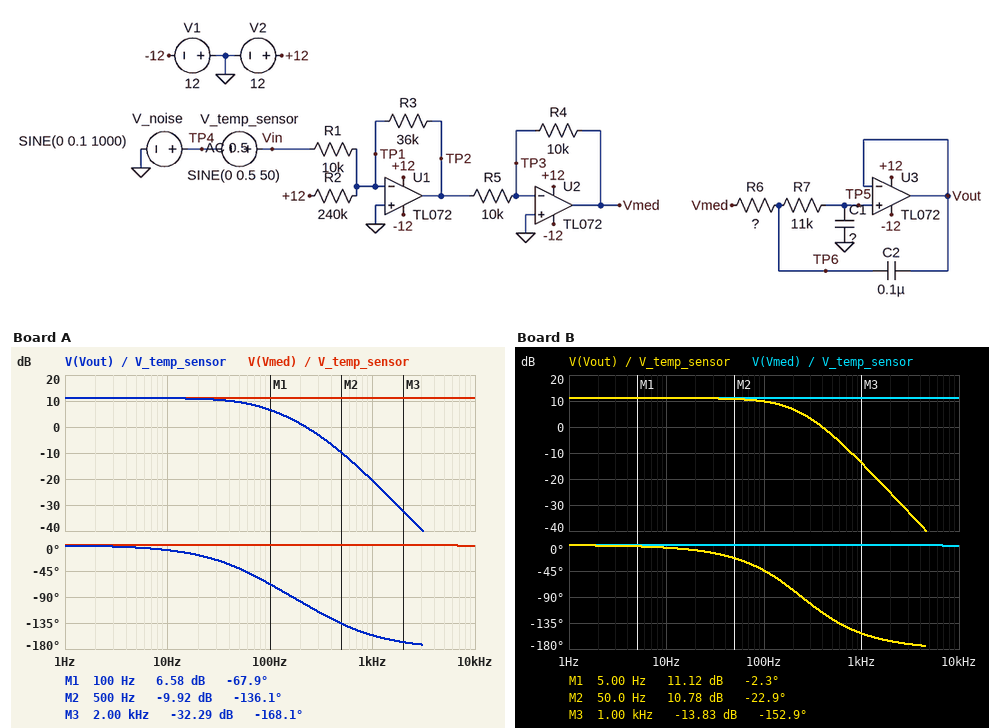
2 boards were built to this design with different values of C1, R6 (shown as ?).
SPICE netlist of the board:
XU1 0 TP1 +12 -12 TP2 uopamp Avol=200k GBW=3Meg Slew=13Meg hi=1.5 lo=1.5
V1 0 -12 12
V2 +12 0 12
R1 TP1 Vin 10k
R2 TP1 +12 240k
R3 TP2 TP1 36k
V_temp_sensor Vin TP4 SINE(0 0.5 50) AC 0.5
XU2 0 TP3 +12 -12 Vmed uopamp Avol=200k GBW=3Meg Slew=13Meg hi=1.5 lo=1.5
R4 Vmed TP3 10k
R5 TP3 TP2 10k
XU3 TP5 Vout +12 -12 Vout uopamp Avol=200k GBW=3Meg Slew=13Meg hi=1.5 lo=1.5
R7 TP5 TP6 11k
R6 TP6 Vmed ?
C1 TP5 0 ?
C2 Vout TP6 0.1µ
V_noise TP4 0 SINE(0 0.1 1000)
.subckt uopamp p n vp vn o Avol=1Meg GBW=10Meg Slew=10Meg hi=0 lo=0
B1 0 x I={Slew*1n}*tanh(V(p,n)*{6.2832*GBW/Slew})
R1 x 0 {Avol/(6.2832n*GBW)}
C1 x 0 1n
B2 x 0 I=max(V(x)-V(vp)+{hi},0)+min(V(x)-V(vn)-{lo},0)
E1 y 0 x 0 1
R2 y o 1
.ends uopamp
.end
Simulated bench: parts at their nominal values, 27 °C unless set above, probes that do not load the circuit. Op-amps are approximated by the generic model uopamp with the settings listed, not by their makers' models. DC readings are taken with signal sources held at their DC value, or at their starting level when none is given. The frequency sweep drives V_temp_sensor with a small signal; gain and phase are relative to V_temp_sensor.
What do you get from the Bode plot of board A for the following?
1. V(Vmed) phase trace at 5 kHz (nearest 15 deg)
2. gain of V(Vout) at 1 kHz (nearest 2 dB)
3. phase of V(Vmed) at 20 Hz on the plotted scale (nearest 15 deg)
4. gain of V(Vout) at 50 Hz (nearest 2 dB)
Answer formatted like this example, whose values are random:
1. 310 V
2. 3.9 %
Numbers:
1. 0 deg
2. -20 dB
3. 0 deg
4. 10 dB
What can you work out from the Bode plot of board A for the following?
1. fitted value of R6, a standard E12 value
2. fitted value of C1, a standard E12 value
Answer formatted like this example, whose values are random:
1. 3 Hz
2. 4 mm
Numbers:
1. 5.6 kΩ
2. 150 nF
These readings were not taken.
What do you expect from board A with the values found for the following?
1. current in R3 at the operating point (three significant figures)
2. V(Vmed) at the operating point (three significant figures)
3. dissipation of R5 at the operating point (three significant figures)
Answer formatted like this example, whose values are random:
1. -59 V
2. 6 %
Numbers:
1. 50.0 µA
2. 1.80 V
3. 324 µW
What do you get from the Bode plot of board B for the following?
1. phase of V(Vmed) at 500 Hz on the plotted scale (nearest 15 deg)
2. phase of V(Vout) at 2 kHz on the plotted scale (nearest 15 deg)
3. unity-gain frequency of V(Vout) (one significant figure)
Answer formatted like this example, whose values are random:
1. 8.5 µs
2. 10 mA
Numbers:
1. 0 deg
2. -165 deg
3. 400 Hz
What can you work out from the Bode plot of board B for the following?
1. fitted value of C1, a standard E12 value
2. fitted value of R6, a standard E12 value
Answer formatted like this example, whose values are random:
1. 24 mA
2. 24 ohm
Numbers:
1. 82 nF
2. 4.7 kΩ
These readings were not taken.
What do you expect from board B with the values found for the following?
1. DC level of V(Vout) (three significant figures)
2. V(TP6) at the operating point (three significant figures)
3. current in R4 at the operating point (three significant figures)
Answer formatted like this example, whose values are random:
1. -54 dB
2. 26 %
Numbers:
1. 1.80 V
2. 1.80 V
3. 180 µA
